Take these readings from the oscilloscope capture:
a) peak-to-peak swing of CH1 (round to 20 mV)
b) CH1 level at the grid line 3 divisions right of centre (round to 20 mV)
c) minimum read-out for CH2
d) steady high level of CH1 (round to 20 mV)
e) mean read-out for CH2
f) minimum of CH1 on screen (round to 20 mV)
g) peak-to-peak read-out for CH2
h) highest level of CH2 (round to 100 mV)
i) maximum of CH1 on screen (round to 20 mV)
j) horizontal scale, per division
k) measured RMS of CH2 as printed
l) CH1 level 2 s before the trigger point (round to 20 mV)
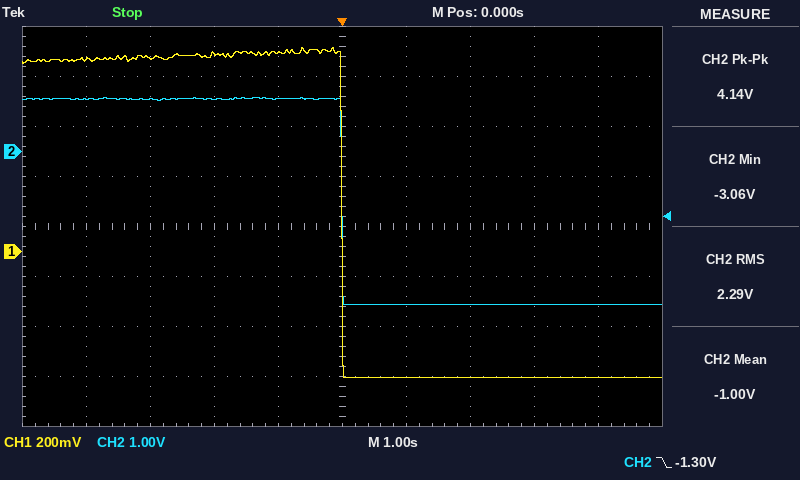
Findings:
1.32 V
-500 mV
-3.06 V
780 mV
-1.00 V
-500 mV
4.14 V
1.1 V
820 mV
1 s
2.29 V
800 mV
